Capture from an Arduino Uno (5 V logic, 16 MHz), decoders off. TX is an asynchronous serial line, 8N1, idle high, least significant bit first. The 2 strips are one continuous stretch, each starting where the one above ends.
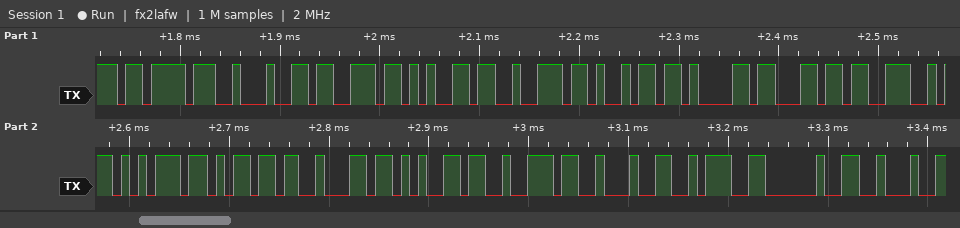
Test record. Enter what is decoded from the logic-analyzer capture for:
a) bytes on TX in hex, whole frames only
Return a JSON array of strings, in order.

["0x7B 0x22 0x73 0x65 0x72 0x69 0x61 0x6C 0x4E 0x75 0x6D 0x62 0x65 0x72 0x22 0x3A 0x20 0x22"]
